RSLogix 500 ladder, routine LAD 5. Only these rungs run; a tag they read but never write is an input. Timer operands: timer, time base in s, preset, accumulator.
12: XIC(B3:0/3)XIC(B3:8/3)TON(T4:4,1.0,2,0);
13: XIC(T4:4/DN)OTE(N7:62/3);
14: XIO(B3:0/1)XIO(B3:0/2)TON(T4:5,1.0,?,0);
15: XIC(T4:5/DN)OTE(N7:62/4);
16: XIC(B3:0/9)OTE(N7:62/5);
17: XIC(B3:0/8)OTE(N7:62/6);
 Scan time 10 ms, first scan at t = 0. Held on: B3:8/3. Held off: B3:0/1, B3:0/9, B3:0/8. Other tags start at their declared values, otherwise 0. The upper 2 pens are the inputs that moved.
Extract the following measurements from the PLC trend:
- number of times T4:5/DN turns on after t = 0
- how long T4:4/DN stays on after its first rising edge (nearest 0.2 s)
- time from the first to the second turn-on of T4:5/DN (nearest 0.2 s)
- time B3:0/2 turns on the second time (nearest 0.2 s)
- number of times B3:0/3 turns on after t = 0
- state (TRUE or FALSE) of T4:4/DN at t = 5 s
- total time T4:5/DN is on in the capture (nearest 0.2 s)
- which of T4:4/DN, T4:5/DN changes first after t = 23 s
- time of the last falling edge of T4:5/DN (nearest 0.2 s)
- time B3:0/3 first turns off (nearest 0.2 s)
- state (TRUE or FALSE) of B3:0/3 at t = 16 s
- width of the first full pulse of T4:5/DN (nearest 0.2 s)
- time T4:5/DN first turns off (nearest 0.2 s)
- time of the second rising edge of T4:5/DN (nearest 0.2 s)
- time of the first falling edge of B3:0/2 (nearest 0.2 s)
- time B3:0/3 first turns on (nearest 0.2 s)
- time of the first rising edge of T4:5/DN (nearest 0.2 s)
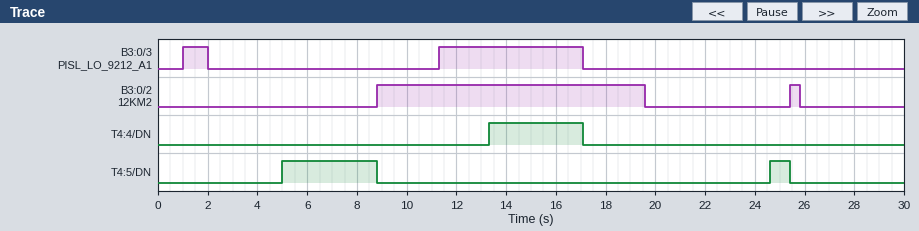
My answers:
2
3.8 s
19.6 s
25.4 s
2
FALSE
4.6 s
T4:5/DN
25.4 s
2.0 s
TRUE
3.8 s
8.8 s
24.6 s
19.6 s
1.0 s
5.0 s
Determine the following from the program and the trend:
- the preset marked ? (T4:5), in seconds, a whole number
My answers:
5 s
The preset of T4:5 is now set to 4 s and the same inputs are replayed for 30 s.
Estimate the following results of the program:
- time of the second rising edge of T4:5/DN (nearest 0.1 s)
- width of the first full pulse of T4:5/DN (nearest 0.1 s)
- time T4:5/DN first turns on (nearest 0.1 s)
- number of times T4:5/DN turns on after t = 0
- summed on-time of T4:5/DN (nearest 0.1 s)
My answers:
23.6 s
4.8 s
4.0 s
3
6.8 s
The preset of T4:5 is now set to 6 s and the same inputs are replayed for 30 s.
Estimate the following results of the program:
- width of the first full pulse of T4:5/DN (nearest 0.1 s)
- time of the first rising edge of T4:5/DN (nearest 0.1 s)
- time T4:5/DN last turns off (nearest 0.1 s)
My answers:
2.8 s
6.0 s
8.8 s
